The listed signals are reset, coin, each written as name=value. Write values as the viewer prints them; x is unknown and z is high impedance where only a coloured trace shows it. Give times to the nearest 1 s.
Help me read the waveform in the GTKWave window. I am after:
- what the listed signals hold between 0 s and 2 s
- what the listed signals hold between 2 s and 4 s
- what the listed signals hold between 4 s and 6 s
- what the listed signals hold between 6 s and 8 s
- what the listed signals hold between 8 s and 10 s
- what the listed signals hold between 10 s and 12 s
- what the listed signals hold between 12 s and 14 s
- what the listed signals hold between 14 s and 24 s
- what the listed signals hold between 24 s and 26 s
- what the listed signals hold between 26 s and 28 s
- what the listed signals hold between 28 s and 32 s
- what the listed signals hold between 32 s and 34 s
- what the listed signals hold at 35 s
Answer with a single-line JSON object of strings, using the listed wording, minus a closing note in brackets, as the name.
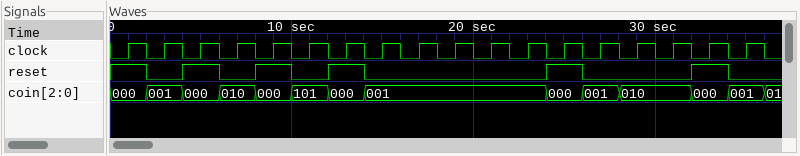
{"what the listed signals hold between 0 s and 2 s": "reset=1, coin=000", "what the listed signals hold between 2 s and 4 s": "reset=0, coin=001", "what the listed signals hold between 4 s and 6 s": "reset=1, coin=000", "what the listed signals hold between 6 s and 8 s": "reset=0, coin=010", "what the listed signals hold between 8 s and 10 s": "reset=1, coin=000", "what the listed signals hold between 10 s and 12 s": "reset=0, coin=101", "what the listed signals hold between 12 s and 14 s": "reset=1, coin=000", "what the listed signals hold between 14 s and 24 s": "reset=0, coin=001", "what the listed signals hold between 24 s and 26 s": "reset=1, coin=000", "what the listed signals hold between 26 s and 28 s": "reset=0, coin=001", "what the listed signals hold between 28 s and 32 s": "reset=0, coin=010", "what the listed signals hold between 32 s and 34 s": "reset=1, coin=000", "what the listed signals hold at 35 s": "reset=0, coin=001"}
